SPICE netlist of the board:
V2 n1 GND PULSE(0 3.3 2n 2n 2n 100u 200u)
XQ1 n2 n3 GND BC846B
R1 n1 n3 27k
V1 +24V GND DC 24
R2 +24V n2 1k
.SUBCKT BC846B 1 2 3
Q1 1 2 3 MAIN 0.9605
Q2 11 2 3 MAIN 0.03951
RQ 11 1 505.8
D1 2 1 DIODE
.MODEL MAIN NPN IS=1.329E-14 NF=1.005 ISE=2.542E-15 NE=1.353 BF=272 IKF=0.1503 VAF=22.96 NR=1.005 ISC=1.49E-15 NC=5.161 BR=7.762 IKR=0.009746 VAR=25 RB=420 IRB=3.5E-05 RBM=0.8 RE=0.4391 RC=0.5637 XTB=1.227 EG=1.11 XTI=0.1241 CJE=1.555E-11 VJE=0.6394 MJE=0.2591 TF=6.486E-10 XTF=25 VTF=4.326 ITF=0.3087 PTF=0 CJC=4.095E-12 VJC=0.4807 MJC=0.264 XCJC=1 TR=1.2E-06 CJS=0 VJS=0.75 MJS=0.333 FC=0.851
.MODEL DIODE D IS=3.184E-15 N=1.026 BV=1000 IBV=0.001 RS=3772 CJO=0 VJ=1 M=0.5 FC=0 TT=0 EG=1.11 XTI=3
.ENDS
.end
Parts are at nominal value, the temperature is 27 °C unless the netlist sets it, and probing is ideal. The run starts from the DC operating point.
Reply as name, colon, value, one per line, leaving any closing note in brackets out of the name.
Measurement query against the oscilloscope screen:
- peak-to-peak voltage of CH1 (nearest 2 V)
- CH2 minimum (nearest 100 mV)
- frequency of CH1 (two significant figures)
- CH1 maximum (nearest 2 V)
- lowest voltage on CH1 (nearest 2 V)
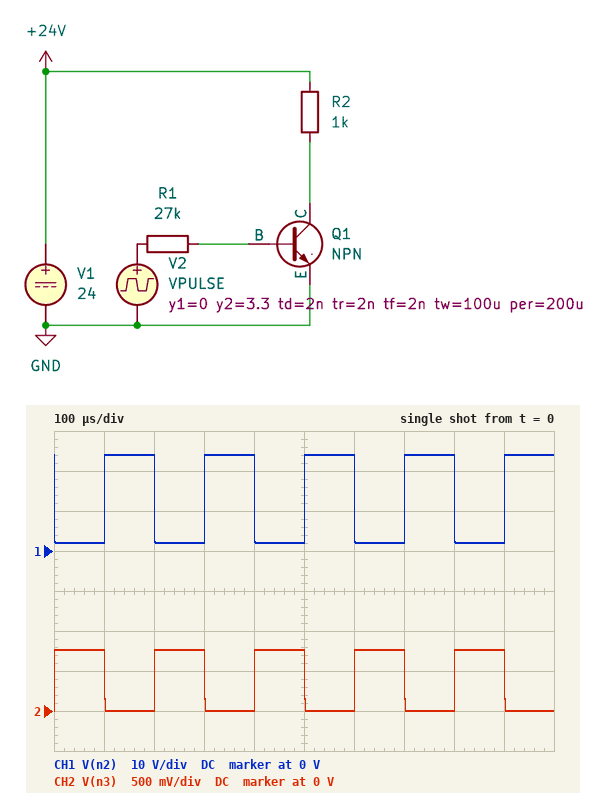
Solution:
peak-to-peak voltage of CH1: 22 V
CH2 minimum: 0 V
frequency of CH1: 5.0 kHz
CH1 maximum: 24 V
lowest voltage on CH1: 2 V
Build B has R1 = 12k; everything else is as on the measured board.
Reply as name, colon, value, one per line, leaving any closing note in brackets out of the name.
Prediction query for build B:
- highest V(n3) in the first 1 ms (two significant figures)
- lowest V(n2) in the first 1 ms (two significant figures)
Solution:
highest V(n3) in the first 1 ms: 780 mV
lowest V(n2) in the first 1 ms: 130 mV
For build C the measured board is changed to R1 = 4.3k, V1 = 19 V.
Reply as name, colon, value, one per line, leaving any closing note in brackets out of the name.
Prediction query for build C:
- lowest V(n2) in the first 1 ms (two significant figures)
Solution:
lowest V(n2) in the first 1 ms: 78 mV
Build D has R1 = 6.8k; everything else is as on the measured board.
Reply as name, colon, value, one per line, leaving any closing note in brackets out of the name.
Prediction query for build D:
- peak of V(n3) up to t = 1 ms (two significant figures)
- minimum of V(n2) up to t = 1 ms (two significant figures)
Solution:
peak of V(n3) up to t = 1 ms: 800 mV
minimum of V(n2) up to t = 1 ms: 110 mV
